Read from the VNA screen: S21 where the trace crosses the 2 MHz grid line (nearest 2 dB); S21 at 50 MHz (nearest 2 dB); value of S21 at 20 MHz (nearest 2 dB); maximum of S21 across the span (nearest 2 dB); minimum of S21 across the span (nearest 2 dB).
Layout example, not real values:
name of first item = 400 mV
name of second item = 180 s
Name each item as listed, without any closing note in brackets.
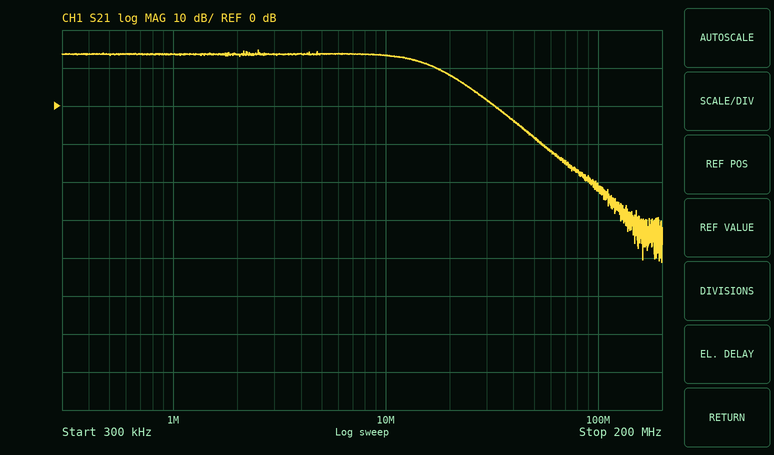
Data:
S21 where the trace crosses the 2 MHz grid line = 14 dB
S21 at 50 MHz = -8 dB
value of S21 at 20 MHz = 8 dB
maximum of S21 across the span = 14 dB
minimum of S21 across the span = -42 dB
